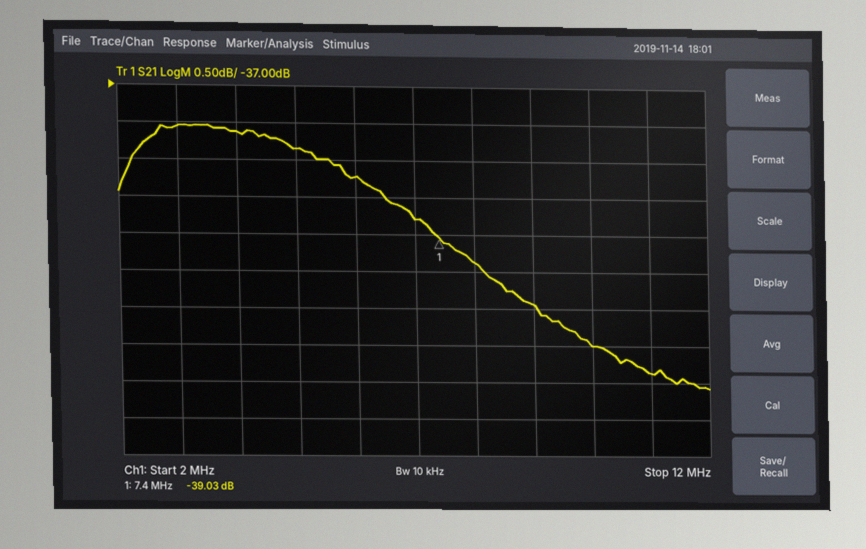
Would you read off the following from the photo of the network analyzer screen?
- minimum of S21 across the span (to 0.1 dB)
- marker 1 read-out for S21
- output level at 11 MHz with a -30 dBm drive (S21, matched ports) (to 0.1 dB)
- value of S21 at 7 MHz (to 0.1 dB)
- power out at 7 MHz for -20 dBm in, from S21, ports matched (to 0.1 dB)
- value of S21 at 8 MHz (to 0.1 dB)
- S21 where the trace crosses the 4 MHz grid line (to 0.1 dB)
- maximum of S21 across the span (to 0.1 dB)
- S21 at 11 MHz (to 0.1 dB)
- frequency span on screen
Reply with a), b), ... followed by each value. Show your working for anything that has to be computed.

a) -41.1 dB
b) -39.03 dB
c) -30 dBm + (-40.9 dB) = -70.9 dBm
d) -38.8 dB
e) -20 dBm + (-38.8 dB) = -58.8 dBm
f) -39.4 dB
g) -37.6 dB
h) -37.5 dB
i) -40.9 dB
j) 10 MHz
